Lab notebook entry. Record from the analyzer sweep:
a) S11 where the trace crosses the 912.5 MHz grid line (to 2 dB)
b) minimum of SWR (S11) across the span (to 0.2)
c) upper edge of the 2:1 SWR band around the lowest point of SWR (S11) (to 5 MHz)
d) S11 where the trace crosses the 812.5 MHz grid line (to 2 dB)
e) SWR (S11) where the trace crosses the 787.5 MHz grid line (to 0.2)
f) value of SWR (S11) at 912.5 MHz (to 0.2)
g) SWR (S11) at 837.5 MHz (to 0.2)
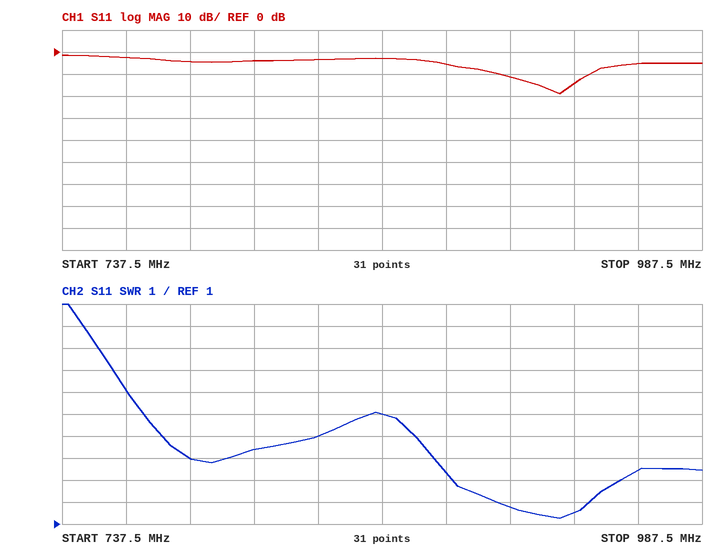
-12 dB
1.2
945 MHz
-4 dB
4.0
1.8
5.0
